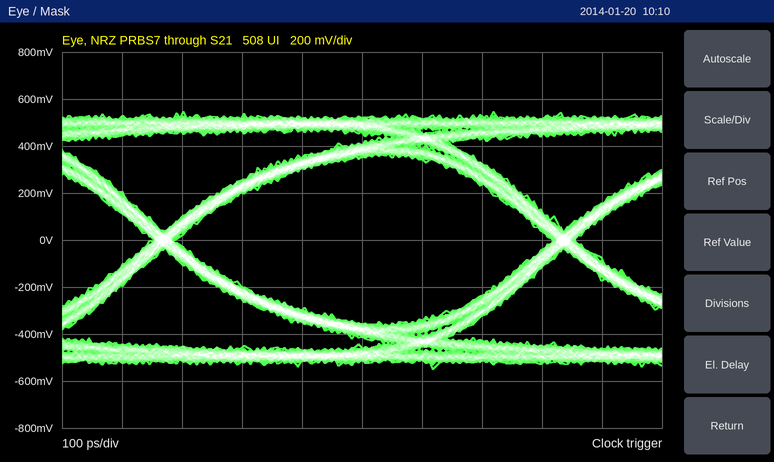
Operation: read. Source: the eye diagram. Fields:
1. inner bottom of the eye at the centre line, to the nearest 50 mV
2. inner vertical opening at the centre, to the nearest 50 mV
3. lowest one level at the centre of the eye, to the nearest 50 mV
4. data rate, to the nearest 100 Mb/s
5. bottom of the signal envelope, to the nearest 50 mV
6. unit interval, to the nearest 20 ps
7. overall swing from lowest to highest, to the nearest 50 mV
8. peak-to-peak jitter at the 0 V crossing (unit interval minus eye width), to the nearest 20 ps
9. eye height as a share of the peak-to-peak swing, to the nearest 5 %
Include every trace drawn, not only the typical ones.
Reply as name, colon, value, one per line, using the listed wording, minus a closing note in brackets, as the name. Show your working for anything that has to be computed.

inner bottom of the eye at the centre line, to the nearest 50 mV: -350 mV
inner vertical opening at the centre, to the nearest 50 mV: 700 mV
lowest one level at the centre of the eye, to the nearest 50 mV: 350 mV
data rate, to the nearest 100 Mb/s: 1.5 Gb/s
bottom of the signal envelope, to the nearest 50 mV: -550 mV
unit interval, to the nearest 20 ps: 660 ps
overall swing from lowest to highest, to the nearest 50 mV: 1.10 V
peak-to-peak jitter at the 0 V crossing (unit interval minus eye width), to the nearest 20 ps: 40 ps
eye height as a share of the peak-to-peak swing, to the nearest 5 %: 700 mV / 1.10 V ≈ 63.6 %, so 65 % to the nearest 5 %
